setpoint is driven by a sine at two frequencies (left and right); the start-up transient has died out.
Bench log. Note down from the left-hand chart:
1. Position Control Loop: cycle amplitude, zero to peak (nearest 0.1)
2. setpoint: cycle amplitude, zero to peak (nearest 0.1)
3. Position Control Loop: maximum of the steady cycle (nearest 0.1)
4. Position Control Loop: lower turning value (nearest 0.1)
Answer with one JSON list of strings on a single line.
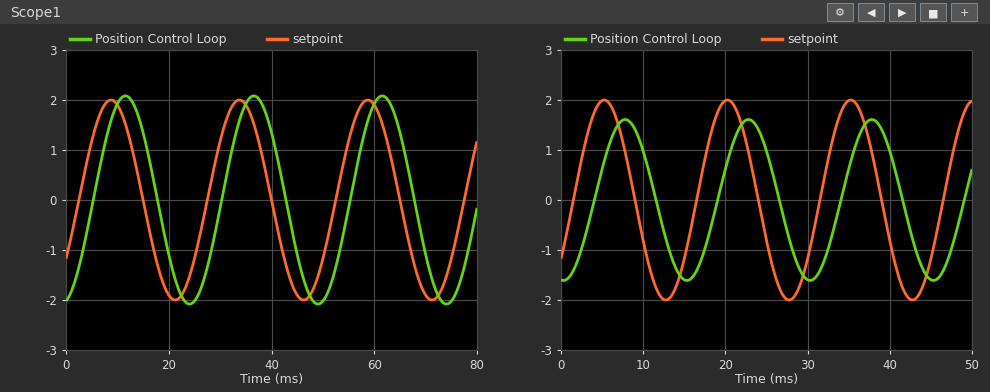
["2.1", "2.0", "2.1", "-2.1"]
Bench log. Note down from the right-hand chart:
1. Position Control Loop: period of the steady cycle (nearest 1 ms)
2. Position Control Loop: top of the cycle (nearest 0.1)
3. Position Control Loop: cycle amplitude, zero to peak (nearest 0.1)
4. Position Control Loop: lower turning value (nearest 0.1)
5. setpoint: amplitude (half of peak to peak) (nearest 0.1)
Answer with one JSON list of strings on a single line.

["15 ms", "1.6", "1.6", "-1.6", "2.0"]
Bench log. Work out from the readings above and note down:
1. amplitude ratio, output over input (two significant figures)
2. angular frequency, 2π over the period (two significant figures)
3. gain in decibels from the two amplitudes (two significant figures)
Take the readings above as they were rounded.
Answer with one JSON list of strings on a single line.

["0.80", "0.42 rad/ms", "-1.9 dB"]
